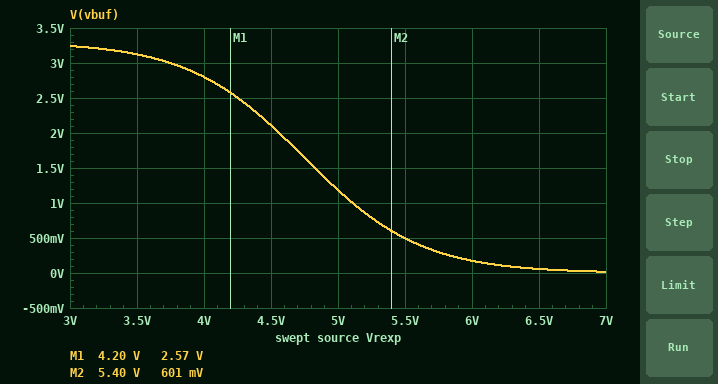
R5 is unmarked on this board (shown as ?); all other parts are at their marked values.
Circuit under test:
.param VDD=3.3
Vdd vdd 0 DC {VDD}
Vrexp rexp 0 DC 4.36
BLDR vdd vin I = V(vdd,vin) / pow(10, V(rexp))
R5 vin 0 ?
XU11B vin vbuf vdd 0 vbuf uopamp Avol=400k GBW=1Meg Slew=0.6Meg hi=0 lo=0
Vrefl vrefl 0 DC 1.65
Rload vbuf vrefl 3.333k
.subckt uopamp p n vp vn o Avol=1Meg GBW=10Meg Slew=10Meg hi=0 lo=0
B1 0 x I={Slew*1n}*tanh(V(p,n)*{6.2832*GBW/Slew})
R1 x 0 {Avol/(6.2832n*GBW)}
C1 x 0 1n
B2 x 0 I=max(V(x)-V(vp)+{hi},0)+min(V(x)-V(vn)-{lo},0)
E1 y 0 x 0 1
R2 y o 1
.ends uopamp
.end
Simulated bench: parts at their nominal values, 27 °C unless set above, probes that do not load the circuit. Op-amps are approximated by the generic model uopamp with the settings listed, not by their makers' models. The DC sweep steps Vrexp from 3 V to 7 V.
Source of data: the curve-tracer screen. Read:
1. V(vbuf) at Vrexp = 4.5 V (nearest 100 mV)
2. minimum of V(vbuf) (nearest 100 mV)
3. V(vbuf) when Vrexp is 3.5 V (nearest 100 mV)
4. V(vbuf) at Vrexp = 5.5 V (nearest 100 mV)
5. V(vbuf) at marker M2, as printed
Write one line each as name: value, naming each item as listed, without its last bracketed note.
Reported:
V(vbuf) at Vrexp = 4.5 V: 2.1 V
minimum of V(vbuf): 0 V
V(vbuf) when Vrexp is 3.5 V: 3.1 V
V(vbuf) at Vrexp = 5.5 V: 500 mV
V(vbuf) at marker M2, as printed: 601 mV
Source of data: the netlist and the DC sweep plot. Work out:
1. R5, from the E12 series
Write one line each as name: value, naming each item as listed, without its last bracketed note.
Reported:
R5, from the E12 series: 56 kΩ
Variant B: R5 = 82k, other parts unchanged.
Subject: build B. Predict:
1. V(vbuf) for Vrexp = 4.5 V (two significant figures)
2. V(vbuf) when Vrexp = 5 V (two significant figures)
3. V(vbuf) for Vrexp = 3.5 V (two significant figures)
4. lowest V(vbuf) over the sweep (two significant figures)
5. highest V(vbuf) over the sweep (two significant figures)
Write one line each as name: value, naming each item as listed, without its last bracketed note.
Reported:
V(vbuf) for Vrexp = 4.5 V: 2.4 V
V(vbuf) when Vrexp = 5 V: 1.5 V
V(vbuf) for Vrexp = 3.5 V: 3.2 V
lowest V(vbuf) over the sweep: 27 mV
highest V(vbuf) over the sweep: 3.3 V
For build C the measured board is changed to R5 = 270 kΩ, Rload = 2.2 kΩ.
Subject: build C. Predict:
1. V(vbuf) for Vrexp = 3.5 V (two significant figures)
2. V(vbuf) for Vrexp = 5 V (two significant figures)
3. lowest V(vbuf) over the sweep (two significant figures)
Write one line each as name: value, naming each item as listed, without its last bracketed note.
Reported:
V(vbuf) for Vrexp = 3.5 V: 3.3 V
V(vbuf) for Vrexp = 5 V: 2.4 V
lowest V(vbuf) over the sweep: 87 mV
